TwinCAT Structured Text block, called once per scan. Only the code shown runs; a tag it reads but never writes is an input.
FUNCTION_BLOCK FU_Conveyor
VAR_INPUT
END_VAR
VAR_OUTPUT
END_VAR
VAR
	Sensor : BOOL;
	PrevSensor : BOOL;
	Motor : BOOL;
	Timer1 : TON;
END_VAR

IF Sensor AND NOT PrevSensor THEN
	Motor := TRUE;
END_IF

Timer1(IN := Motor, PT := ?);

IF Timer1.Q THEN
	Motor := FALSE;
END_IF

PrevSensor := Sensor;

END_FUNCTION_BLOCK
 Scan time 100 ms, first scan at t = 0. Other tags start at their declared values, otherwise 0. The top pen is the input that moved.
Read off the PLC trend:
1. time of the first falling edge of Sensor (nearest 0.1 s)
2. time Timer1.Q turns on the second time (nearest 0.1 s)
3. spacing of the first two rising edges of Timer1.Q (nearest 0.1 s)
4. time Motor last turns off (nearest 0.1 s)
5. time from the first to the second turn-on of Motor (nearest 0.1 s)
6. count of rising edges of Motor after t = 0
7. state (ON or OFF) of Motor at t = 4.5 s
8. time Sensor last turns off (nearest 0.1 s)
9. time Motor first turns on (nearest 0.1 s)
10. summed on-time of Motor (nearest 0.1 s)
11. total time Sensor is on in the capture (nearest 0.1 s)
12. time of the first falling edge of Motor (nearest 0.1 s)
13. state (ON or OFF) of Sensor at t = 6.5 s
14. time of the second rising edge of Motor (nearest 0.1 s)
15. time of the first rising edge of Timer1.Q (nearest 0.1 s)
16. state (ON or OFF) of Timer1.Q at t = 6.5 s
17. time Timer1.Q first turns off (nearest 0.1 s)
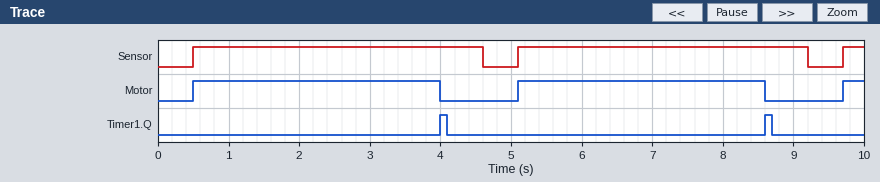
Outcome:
4.6 s
8.6 s
4.6 s
8.6 s
4.6 s
3
OFF
9.2 s
0.5 s
7.3 s
8.5 s
4.0 s
ON
5.1 s
4.0 s
OFF
4.1 s
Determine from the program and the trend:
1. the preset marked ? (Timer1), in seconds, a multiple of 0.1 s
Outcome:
3.5 s
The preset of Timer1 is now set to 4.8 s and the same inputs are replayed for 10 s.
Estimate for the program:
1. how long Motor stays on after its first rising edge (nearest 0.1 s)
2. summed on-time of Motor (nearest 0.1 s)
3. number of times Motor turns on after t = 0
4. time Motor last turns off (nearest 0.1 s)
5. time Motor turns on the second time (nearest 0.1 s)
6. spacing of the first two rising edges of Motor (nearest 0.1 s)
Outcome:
4.8 s
5.1 s
2
5.3 s
9.7 s
9.2 s
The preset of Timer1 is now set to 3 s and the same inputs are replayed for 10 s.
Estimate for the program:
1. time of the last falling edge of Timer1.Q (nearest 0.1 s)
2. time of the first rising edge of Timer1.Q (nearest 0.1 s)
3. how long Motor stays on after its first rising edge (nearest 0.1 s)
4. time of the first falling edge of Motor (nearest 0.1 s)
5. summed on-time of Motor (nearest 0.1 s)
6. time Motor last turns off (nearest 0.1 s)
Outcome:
8.2 s
3.5 s
3.0 s
3.5 s
6.3 s
8.1 s
